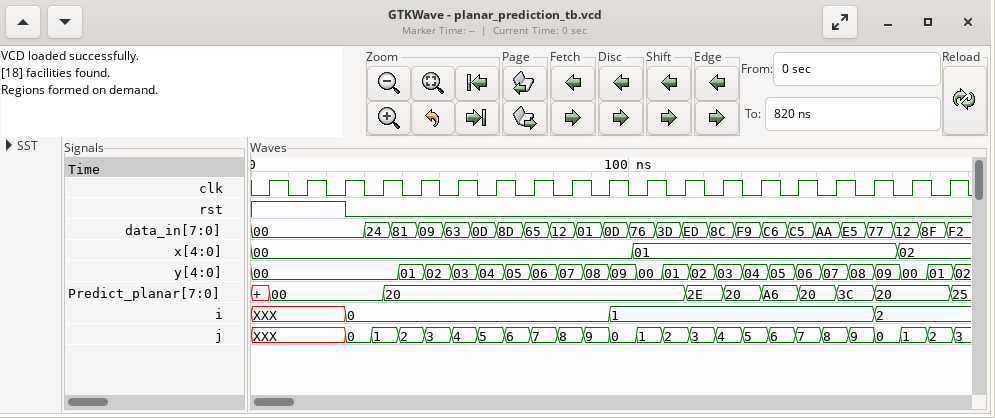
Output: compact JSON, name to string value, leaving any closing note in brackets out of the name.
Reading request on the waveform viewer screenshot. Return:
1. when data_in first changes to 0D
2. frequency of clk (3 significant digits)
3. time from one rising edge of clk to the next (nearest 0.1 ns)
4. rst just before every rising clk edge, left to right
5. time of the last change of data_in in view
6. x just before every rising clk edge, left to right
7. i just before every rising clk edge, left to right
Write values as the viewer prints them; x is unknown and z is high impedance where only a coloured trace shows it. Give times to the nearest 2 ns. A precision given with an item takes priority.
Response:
{"when data_in first changes to 0D": "58 ns", "frequency of clk": "100 MHz", "time from one rising edge of clk to the next": "10 ns", "rst just before every rising clk edge, left to right": "1 1 1 0 0 0 0 0 0 0 0 0 0 0 0 0 0 0 0", "time of the last change of data_in in view": "184 ns", "x just before every rising clk edge, left to right": "00, 00, 00, 00, 00, 00, 00, 00, 00, 00, 01, 01, 01, 01, 01, 01, 01, 02, 02", "i just before every rising clk edge, left to right": "XXX, XXX, XXX, 0, 0, 0, 0, 0, 0, 0, 1, 1, 1, 1, 1, 1, 1, 2, 2"}
